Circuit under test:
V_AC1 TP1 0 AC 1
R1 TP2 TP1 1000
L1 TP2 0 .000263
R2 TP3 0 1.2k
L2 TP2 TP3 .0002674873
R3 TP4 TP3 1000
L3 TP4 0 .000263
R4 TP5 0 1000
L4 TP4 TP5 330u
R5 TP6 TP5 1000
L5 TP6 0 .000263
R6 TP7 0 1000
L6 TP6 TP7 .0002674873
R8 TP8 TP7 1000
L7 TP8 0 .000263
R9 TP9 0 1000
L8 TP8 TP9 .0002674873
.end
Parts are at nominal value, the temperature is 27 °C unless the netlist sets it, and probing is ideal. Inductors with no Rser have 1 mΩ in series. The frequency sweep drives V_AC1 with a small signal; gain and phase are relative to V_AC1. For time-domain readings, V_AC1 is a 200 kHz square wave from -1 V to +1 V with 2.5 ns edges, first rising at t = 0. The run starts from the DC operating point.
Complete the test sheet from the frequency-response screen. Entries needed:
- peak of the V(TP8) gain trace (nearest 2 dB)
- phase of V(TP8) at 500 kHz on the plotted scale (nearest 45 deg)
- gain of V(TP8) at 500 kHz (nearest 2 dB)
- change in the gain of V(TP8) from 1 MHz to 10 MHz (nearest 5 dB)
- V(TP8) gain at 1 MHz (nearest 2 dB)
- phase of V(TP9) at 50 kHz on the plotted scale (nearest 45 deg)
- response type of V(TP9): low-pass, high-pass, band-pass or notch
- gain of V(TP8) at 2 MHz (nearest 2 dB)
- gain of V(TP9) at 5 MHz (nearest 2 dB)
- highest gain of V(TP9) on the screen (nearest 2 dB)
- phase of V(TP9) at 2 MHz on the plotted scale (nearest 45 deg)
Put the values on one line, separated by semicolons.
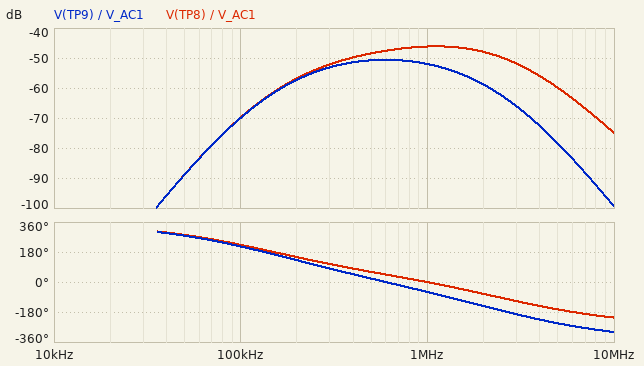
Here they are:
-46 dB; 45 deg; -48 dB; -30 dB; -46 dB; 270 deg; band-pass; -48 dB; -78 dB; -50 dB; -135 deg
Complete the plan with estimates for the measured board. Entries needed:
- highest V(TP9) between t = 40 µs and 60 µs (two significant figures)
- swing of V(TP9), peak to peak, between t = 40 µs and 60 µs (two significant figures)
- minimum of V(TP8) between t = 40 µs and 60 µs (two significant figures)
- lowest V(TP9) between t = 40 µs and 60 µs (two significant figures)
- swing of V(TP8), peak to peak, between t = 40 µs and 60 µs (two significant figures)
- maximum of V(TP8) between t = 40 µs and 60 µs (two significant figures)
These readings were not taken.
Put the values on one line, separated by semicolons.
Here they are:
3.1 mV; 6.2 mV; -6.0 mV; -3.1 mV; 12 mV; 6.0 mV
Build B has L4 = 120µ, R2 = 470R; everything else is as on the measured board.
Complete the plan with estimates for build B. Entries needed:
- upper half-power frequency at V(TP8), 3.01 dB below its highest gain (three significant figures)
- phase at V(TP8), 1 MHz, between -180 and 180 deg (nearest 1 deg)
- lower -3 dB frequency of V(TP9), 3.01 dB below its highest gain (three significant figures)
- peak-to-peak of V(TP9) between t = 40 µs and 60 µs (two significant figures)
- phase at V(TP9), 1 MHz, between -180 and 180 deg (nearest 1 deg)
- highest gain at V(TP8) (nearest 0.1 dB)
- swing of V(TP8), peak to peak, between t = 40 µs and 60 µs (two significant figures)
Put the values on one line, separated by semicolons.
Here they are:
2.38 MHz; 1 deg; 284 kHz; 5.7 mV; -58 deg; -47.0 dB; 11 mV
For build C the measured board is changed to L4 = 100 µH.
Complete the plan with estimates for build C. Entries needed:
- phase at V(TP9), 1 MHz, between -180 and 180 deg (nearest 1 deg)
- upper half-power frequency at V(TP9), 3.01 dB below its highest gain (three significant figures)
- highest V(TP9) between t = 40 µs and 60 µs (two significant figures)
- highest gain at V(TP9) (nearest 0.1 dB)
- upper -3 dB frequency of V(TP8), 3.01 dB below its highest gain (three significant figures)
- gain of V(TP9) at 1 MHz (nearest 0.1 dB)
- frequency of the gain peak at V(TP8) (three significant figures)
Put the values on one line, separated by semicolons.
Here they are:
-45 deg; 1.40 MHz; 4.4 mV; -47.0 dB; 2.69 MHz; -47.9 dB; 1.28 MHz
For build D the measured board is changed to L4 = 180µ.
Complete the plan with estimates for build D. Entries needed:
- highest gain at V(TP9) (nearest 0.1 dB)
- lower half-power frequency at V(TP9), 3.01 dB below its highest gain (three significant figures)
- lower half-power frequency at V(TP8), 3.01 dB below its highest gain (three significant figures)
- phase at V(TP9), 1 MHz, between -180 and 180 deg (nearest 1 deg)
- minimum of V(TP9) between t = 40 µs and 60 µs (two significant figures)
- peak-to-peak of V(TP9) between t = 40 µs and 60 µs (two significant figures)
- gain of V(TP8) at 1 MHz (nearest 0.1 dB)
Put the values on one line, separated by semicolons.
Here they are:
-48.4 dB; 298 kHz; 486 kHz; -52 deg; -3.9 mV; 7.7 mV; -43.7 dB
